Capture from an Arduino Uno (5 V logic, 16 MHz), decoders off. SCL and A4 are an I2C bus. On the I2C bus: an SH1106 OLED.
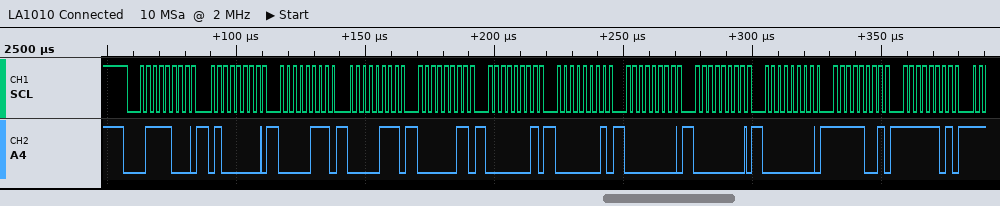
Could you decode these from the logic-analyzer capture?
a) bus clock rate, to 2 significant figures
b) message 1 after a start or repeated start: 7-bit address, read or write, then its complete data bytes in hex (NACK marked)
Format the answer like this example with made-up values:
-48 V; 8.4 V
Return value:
400 kHz; 0x3C write: 40 07 07 03 01 01 00 00 00 F9 FD
